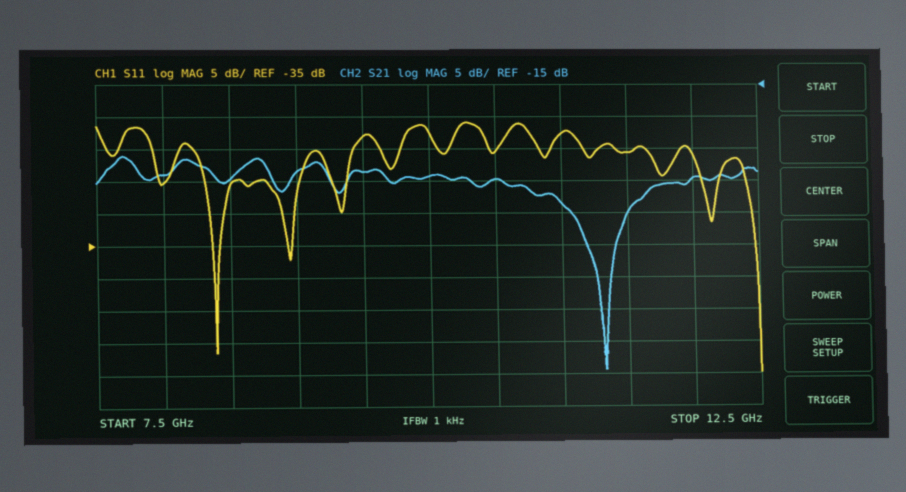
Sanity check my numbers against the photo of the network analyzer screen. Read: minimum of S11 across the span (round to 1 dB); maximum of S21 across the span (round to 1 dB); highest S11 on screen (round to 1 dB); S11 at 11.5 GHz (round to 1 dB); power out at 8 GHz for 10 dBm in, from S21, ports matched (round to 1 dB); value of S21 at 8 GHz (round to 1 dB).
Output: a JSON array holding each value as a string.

["-55 dB", "-26 dB", "-16 dB", "-21 dB", "-19 dBm", "-29 dB"]
